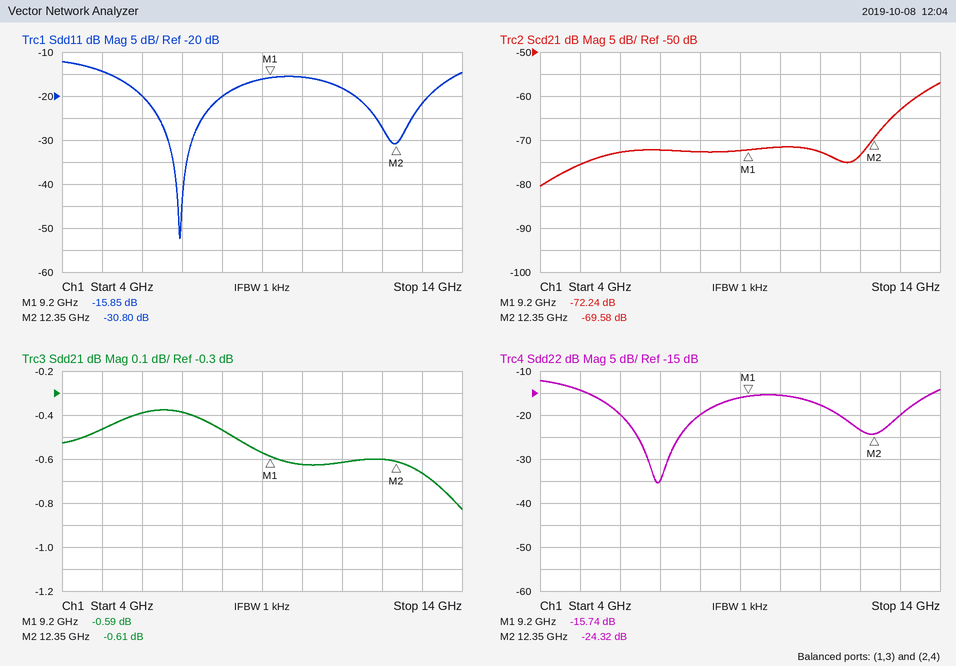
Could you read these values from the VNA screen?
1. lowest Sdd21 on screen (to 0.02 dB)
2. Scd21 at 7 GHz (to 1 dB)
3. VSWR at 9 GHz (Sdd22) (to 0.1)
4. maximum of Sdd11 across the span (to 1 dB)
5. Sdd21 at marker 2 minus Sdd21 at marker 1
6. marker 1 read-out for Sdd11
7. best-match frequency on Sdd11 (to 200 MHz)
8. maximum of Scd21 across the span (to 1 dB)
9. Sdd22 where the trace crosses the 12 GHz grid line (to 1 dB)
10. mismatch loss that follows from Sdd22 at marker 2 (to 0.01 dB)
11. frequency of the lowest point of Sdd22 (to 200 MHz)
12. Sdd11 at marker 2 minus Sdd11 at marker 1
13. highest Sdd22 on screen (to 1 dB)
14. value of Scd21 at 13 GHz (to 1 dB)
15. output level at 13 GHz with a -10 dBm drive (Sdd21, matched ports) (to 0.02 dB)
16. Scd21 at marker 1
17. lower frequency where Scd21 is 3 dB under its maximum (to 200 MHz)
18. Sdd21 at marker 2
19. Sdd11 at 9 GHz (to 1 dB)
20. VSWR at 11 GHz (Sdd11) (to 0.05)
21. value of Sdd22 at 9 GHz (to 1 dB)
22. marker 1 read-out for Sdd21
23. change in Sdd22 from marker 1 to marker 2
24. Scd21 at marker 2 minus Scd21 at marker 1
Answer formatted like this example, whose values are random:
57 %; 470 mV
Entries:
-0.82 dB; -72 dB; 1.4; -12 dB; -0.02 dB; -15.85 dB; 7.0 GHz; -57 dB; -23 dB; 0.02 dB; 7.0 GHz; -14.95 dB; -12 dB; -63 dB; -10.66 dBm; -72.24 dB; 13.4 GHz; -0.61 dB; -16 dB; 1.30; -16 dB; -0.59 dB; -8.58 dB; 2.66 dB
